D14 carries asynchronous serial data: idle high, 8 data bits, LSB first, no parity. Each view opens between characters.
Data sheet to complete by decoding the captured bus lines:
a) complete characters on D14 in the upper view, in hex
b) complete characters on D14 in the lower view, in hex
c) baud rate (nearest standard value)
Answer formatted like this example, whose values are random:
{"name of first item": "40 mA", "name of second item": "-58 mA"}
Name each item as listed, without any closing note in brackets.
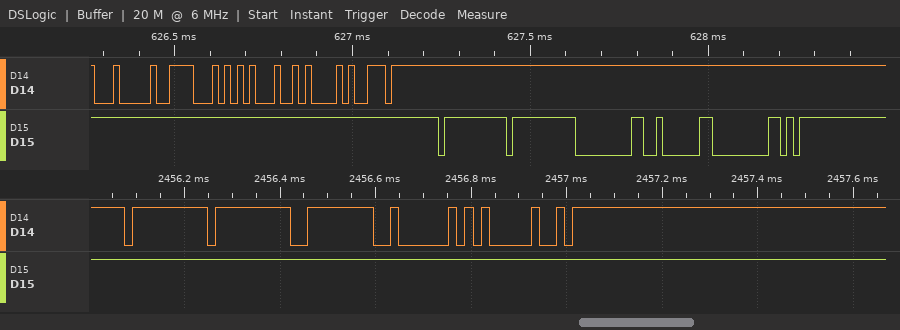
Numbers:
{"complete characters on D14 in the upper view, in hex": "04, 1E, 15, 0A, B9", "complete characters on D14 in the lower view, in hex": "FF, FF, FE, 02, 05, FA", "baud rate": "57600 baud"}
